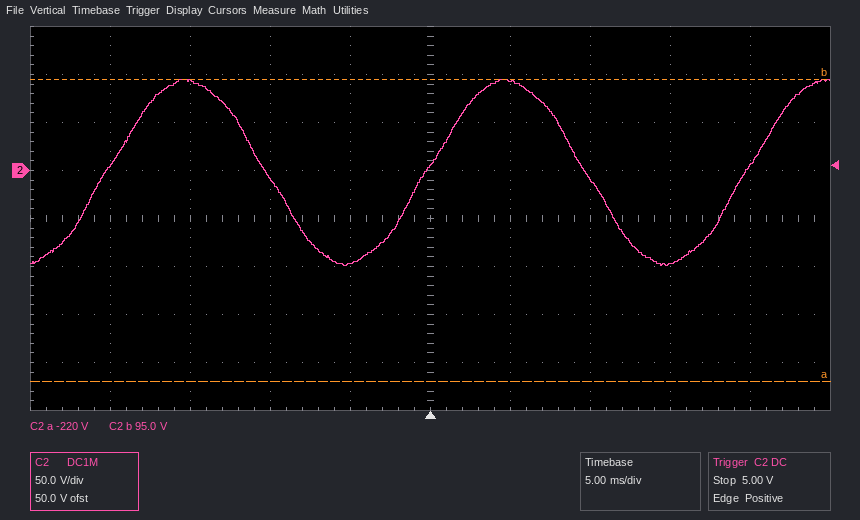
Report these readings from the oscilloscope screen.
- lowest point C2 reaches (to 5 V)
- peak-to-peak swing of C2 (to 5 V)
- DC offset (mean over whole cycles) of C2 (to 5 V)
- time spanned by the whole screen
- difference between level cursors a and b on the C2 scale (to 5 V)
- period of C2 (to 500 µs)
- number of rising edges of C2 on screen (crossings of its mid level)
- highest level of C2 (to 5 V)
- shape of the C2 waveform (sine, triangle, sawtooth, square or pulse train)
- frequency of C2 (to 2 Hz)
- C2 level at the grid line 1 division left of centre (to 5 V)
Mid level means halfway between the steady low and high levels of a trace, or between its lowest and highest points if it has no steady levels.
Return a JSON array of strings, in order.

["-100 V", "195 V", "0 V", "50 ms", "315 V", "20.0 ms", "3", "95 V", "sine", "50 Hz", "-95 V"]
